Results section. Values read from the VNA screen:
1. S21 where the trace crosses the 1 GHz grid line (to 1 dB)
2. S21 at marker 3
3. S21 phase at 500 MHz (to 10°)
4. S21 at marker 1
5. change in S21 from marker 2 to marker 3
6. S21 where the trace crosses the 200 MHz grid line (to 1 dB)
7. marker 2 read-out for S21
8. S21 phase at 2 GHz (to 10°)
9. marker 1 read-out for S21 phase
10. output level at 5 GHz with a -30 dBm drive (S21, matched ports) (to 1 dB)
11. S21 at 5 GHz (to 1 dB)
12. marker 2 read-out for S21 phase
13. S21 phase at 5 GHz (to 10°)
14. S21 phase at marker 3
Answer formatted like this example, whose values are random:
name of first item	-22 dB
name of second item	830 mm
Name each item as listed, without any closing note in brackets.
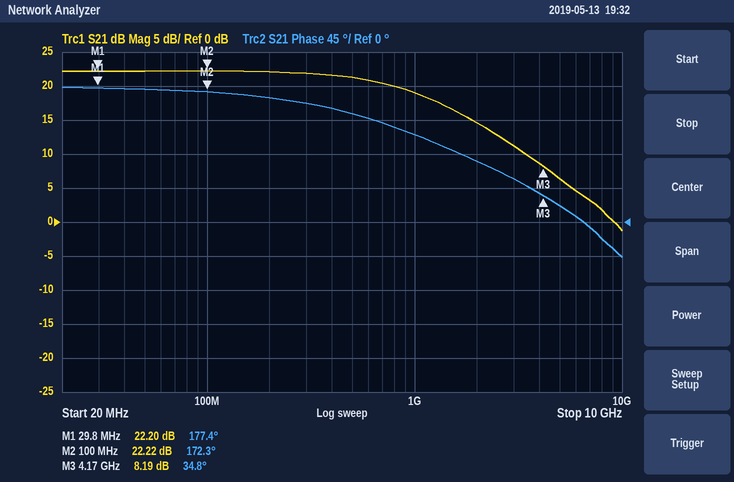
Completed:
S21 where the trace crosses the 1 GHz grid line	19 dB
S21 at marker 3	8.19 dB
S21 phase at 500 MHz	140°
S21 at marker 1	22.20 dB
change in S21 from marker 2 to marker 3	-14.03 dB
S21 where the trace crosses the 200 MHz grid line	22 dB
marker 2 read-out for S21	22.22 dB
S21 phase at 2 GHz	80°
marker 1 read-out for S21 phase	177.4°
output level at 5 GHz with a -30 dBm drive (S21, matched ports)	-24 dBm
S21 at 5 GHz	6 dB
marker 2 read-out for S21 phase	172.3°
S21 phase at 5 GHz	20°
S21 phase at marker 3	34.8°
